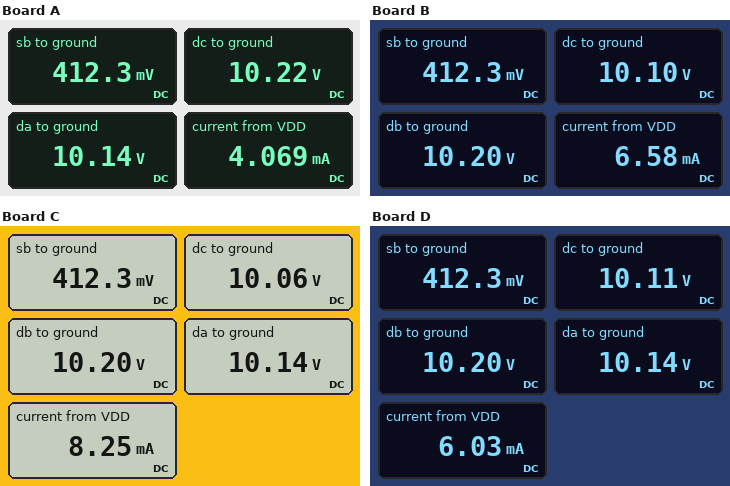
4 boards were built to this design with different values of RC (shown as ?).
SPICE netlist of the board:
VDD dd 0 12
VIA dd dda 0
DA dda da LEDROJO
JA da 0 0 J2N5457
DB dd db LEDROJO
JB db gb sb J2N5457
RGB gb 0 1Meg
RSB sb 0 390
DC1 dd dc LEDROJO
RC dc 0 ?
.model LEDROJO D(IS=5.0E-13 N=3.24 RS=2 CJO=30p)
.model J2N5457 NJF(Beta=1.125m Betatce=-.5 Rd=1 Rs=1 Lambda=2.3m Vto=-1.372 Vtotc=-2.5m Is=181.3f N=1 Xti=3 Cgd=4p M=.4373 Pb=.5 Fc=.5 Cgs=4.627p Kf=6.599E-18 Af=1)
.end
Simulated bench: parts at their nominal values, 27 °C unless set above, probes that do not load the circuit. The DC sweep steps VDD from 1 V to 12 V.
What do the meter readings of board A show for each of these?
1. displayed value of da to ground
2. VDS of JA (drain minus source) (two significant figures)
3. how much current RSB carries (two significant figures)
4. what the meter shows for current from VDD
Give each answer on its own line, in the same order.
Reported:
10.14 V
10 V
1.1 mA
4.069 mA
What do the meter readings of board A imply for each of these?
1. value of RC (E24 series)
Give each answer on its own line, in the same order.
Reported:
12 kΩ
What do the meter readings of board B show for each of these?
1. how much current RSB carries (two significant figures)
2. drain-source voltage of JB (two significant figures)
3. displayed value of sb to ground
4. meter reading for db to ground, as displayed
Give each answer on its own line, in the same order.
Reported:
1.1 mA
9.8 V
412.3 mV
10.20 V
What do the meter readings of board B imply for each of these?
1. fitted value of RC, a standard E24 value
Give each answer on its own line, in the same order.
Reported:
3 kΩ
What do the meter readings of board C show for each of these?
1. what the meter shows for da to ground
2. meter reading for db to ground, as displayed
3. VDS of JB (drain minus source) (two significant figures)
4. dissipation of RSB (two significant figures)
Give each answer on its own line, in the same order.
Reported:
10.14 V
10.20 V
9.8 V
440 µW
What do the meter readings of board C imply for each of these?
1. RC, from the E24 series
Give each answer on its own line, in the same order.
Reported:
2 kΩ
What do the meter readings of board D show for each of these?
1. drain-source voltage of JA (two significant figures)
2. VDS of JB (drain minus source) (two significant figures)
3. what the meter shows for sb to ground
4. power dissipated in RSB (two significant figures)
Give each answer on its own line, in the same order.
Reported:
10 V
9.8 V
412.3 mV
440 µW
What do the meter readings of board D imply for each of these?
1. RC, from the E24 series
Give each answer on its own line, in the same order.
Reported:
3.6 kΩ
